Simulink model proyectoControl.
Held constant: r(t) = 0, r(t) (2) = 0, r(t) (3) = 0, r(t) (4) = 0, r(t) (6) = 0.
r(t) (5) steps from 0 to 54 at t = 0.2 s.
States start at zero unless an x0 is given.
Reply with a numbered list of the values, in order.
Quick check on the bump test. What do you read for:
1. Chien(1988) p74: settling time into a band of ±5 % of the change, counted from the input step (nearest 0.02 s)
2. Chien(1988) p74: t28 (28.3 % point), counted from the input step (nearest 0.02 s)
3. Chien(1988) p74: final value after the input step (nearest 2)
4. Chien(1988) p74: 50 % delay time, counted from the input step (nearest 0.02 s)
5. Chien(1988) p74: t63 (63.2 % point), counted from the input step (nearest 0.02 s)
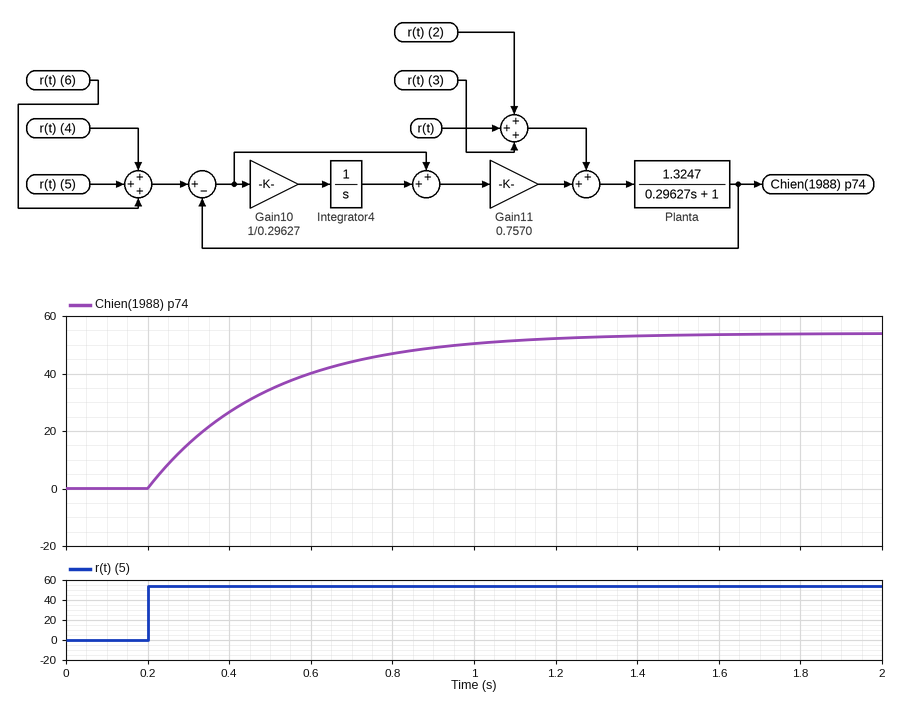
1. 0.88 s
2. 0.10 s
3. 54
4. 0.20 s
5. 0.30 s
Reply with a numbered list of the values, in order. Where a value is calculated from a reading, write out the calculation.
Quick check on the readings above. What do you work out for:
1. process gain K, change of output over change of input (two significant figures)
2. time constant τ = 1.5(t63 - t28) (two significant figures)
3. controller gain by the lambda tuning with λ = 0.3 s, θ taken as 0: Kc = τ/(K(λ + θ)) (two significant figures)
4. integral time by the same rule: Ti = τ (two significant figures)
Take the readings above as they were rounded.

1. (54 - 0) / 54 = 1.0
2. 1.5 × (0.3 - 0.1) = 0.30 s
3. 0.3 / (1 × (0.3 + 0)) = 1.0
4. 0.30 s
